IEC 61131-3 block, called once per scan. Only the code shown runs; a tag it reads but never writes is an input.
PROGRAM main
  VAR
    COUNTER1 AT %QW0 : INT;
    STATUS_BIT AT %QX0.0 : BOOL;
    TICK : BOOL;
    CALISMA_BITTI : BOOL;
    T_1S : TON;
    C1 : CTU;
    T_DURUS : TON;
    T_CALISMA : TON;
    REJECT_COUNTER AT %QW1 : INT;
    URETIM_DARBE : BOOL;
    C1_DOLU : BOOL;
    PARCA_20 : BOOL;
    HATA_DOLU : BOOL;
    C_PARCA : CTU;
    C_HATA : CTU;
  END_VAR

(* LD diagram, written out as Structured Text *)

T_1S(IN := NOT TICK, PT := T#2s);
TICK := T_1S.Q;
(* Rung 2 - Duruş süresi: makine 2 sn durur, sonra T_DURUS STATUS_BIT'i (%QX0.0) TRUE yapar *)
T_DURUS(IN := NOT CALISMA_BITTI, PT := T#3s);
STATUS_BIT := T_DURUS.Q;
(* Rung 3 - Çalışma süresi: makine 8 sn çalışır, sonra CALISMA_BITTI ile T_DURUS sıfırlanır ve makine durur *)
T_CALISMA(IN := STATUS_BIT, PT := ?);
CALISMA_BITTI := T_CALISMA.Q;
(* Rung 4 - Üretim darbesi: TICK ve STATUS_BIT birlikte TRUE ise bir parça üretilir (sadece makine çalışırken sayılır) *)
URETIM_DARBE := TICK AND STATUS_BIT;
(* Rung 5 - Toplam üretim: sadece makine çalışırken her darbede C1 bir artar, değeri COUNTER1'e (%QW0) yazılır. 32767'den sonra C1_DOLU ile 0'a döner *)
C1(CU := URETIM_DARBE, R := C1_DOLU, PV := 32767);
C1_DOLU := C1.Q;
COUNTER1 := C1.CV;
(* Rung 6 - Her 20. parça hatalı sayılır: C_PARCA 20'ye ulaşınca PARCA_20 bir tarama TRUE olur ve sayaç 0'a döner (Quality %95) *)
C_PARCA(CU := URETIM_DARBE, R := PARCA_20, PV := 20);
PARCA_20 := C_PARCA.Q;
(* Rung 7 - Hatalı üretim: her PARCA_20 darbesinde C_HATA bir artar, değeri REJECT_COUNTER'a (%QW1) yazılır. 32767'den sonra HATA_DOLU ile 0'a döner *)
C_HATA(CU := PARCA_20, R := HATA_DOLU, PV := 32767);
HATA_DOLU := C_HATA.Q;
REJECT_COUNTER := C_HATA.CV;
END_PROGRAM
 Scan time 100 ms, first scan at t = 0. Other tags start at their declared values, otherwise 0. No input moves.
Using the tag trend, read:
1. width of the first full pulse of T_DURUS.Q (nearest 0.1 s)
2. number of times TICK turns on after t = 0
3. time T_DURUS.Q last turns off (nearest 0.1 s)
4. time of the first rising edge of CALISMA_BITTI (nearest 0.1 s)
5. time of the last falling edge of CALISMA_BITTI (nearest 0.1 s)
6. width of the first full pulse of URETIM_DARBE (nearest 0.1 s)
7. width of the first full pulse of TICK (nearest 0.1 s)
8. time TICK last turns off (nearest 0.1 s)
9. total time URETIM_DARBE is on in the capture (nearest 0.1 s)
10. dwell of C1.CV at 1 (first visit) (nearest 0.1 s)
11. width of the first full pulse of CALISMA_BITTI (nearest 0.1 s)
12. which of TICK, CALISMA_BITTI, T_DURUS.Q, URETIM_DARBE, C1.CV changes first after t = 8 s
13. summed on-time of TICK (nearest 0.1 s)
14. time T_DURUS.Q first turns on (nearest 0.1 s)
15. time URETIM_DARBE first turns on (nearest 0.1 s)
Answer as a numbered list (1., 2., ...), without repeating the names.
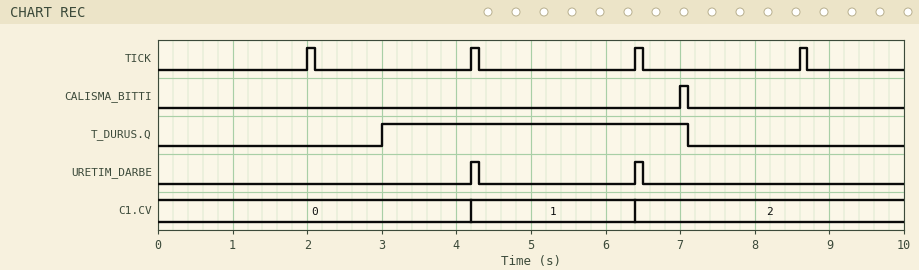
1. 4.1 s
2. 4
3. 7.1 s
4. 7.0 s
5. 7.1 s
6. 0.1 s
7. 0.1 s
8. 8.7 s
9. 0.2 s
10. 2.2 s
11. 0.1 s
12. TICK
13. 0.4 s
14. 3.0 s
15. 4.2 s
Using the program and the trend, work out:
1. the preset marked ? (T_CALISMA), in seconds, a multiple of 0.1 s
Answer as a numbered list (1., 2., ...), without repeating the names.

1. 4.0 s
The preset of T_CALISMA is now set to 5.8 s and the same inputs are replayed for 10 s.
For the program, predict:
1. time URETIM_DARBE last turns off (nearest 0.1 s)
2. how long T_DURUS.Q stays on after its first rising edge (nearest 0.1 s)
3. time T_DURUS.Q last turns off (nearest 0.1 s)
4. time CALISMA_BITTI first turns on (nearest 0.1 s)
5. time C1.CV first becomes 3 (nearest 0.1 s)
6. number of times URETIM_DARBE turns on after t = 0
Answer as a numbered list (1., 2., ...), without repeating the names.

1. 8.7 s
2. 5.9 s
3. 8.9 s
4. 8.8 s
5. 8.6 s
6. 3
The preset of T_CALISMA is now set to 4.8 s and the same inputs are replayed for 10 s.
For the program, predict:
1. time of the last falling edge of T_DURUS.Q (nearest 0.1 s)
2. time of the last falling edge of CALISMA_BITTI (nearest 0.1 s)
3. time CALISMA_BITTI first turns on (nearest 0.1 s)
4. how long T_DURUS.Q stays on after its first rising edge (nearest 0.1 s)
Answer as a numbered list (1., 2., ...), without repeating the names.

1. 7.9 s
2. 7.9 s
3. 7.8 s
4. 4.9 s
